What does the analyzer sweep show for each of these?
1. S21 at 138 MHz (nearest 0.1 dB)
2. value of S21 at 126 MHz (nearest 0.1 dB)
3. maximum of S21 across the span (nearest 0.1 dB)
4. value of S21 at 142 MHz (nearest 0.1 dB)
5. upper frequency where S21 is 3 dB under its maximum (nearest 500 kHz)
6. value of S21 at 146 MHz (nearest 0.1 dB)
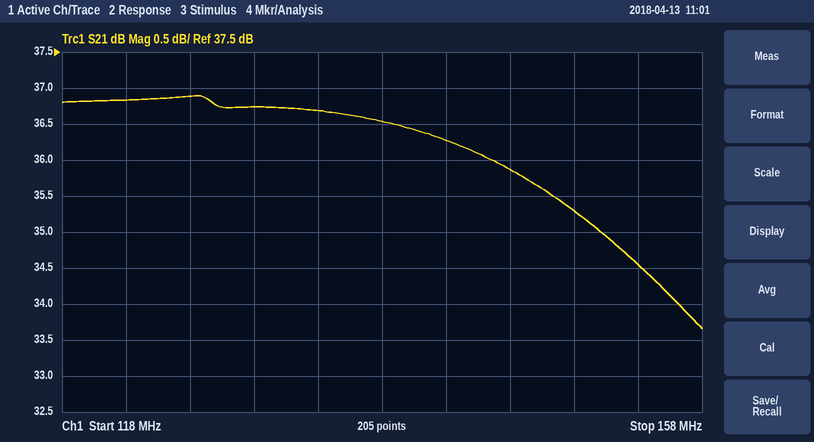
36.5 dB
36.9 dB
36.9 dB
36.3 dB
157.0 MHz
35.9 dB
